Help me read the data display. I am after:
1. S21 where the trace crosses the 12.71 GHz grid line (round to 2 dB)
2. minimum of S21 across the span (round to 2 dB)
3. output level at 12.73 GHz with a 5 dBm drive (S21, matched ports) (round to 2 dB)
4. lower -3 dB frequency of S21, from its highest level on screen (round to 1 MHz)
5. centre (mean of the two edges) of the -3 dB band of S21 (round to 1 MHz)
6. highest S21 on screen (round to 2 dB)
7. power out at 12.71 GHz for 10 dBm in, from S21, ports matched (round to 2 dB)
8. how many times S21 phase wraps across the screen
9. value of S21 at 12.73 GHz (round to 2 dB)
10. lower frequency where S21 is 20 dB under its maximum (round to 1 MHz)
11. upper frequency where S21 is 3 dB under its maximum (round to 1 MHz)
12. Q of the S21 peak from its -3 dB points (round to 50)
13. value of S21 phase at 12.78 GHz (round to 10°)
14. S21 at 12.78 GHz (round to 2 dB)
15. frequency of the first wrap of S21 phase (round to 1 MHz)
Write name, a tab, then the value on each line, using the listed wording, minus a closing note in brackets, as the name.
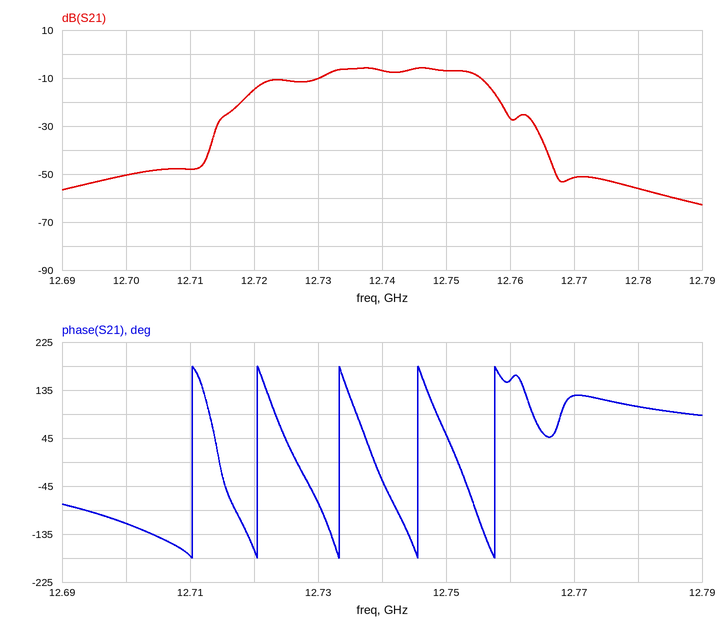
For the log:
S21 where the trace crosses the 12.71 GHz grid line	-48 dB
minimum of S21 across the span	-62 dB
output level at 12.73 GHz with a 5 dBm drive (S21, matched ports)	-6 dBm
lower -3 dB frequency of S21, from its highest level on screen	12.731 GHz
centre (mean of the two edges) of the -3 dB band of S21	12.743 GHz
highest S21 on screen	-6 dB
power out at 12.71 GHz for 10 dBm in, from S21, ports matched	-38 dBm
how many times S21 phase wraps across the screen	5
value of S21 at 12.73 GHz	-10 dB
lower frequency where S21 is 20 dB under its maximum	12.715 GHz
upper frequency where S21 is 3 dB under its maximum	12.755 GHz
Q of the S21 peak from its -3 dB points	550
value of S21 phase at 12.78 GHz	100°
S21 at 12.78 GHz	-56 dB
frequency of the first wrap of S21 phase	12.710 GHz
